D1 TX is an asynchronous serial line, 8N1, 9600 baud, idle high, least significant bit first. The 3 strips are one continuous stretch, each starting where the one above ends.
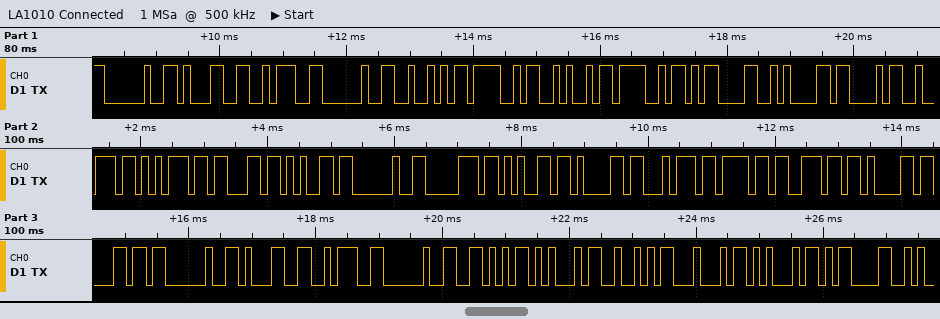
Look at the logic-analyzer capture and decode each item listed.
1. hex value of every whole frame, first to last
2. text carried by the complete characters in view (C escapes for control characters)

20 31 3A 20 52 4F 4A 4F 0D 0A 43 72 75 63 65 20 70 65 61 74 6F 6E 61 6C 20 31 3A 20 56 45 52 44 45 0D
" 1: ROJO\r\nCruce peatonal 1: VERDE\r"
